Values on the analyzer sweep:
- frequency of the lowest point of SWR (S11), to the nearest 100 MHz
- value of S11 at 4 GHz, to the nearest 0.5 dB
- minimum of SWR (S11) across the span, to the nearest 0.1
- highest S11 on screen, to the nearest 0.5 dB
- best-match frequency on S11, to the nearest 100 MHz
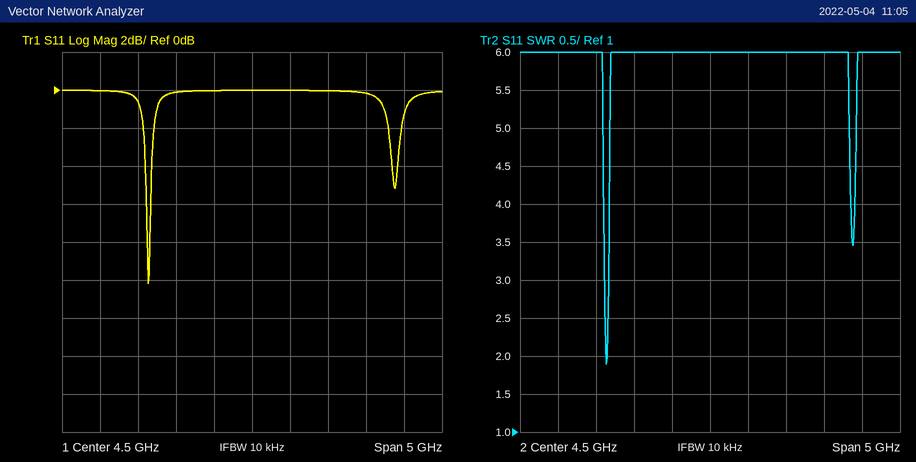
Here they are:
3.1 GHz
0.0 dB
1.9
0.0 dB
3.1 GHz
